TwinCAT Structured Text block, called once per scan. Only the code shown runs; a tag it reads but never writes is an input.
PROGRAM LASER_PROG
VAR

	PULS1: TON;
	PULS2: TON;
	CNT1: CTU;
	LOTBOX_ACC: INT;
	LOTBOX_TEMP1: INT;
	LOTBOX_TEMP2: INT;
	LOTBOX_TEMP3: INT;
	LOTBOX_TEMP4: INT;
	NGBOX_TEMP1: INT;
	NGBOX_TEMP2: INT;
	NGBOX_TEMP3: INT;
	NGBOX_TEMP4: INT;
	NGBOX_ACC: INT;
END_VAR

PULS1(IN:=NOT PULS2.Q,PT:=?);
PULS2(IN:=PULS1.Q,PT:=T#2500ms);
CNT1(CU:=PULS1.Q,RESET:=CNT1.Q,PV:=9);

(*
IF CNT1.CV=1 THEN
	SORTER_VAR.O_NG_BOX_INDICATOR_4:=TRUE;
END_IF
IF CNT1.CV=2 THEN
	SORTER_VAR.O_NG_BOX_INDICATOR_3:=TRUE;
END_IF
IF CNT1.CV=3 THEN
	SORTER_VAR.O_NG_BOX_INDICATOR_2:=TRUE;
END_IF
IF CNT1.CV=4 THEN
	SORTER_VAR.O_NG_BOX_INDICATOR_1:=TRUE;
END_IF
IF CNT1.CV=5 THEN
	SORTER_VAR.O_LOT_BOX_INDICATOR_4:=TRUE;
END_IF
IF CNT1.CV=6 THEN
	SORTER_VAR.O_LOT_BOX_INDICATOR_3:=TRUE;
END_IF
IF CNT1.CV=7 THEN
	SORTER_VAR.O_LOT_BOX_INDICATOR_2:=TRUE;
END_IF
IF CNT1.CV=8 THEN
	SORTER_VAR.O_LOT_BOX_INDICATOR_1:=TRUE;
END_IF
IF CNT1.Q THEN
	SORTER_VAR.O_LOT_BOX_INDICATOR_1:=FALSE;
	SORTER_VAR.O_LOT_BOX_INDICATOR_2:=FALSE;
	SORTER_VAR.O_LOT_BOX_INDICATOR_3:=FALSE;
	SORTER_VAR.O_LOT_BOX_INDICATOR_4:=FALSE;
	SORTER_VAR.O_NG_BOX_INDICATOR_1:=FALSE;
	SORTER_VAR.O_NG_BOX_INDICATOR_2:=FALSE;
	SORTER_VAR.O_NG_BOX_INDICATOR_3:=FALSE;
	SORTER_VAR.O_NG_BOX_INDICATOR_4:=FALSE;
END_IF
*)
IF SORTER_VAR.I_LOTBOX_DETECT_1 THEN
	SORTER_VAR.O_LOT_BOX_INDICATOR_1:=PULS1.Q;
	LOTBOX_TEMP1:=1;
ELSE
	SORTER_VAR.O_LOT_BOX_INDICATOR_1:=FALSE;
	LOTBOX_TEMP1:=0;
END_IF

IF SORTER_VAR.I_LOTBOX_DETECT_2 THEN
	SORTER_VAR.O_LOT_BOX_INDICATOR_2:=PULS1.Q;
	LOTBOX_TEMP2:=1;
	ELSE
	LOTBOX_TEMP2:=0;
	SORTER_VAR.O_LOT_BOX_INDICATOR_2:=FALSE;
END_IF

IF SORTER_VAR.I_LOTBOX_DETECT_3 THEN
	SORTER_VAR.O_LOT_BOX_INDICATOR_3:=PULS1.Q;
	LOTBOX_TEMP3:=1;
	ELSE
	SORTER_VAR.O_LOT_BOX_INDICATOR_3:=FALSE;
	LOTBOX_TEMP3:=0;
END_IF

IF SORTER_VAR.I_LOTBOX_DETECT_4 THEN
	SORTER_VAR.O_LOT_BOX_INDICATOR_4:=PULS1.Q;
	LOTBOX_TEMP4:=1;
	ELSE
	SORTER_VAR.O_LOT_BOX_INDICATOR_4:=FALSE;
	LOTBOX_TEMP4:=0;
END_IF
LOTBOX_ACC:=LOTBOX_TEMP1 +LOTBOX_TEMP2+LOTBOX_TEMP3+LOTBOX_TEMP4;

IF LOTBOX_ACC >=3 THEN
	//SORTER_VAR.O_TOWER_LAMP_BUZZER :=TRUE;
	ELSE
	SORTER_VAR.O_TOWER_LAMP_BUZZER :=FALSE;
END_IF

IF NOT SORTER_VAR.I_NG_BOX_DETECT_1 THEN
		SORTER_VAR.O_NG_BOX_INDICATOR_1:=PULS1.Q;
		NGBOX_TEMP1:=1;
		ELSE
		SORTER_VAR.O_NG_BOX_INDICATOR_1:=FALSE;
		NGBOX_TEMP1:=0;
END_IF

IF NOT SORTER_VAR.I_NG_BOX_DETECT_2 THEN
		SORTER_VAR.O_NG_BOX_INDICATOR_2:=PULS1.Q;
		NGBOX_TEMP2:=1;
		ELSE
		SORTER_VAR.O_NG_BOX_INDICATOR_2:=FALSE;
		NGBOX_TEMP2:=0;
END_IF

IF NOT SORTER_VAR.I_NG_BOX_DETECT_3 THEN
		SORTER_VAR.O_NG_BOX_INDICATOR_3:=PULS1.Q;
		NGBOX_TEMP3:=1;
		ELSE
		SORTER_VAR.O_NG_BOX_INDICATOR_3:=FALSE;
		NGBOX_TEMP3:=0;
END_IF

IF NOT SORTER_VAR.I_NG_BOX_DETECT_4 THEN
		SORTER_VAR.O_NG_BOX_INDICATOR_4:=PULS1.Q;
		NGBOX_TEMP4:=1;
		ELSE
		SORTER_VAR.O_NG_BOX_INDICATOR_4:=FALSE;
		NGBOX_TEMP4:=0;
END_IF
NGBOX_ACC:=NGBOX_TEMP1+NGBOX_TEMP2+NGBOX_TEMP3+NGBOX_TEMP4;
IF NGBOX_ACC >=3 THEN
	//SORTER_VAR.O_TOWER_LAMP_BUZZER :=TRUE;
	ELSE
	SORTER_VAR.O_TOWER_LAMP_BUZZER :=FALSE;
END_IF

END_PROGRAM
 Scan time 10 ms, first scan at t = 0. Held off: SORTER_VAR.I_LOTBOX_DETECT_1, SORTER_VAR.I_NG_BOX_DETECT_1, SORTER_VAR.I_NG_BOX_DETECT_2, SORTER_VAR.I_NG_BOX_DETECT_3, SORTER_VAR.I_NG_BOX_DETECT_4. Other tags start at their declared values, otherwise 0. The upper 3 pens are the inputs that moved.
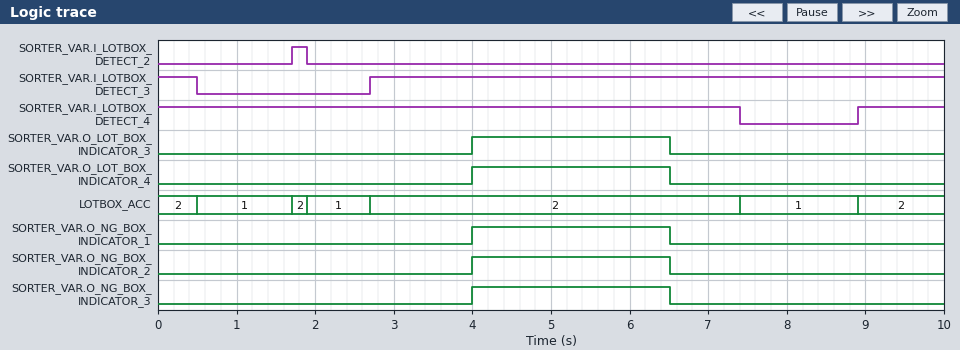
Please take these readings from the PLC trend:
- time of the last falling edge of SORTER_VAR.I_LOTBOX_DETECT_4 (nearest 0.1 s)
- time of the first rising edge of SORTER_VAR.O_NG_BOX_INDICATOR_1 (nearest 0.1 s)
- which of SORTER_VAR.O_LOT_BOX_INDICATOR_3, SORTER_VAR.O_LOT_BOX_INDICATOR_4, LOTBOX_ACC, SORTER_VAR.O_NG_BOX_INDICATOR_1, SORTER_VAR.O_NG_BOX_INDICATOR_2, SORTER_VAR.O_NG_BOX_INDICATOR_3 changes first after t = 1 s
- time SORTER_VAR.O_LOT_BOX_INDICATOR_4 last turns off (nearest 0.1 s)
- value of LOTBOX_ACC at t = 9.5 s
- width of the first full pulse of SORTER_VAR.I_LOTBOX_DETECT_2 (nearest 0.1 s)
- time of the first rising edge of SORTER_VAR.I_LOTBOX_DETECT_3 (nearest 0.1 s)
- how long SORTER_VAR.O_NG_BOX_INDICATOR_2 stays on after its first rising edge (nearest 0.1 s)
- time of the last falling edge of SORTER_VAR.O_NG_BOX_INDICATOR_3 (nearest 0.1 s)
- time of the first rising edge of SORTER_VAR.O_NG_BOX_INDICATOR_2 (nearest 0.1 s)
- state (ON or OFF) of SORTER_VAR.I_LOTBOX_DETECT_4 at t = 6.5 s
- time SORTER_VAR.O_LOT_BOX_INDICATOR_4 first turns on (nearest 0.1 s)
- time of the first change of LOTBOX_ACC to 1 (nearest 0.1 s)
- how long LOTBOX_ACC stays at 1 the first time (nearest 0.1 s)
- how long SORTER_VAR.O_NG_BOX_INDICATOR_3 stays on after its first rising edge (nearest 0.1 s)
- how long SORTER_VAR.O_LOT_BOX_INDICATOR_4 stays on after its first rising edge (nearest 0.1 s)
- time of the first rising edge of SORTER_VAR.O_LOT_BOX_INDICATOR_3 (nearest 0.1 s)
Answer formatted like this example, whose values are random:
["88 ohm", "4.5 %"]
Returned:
["7.4 s", "4.0 s", "LOTBOX_ACC", "6.5 s", "2", "0.2 s", "2.7 s", "2.5 s", "6.5 s", "4.0 s", "ON", "4.0 s", "0.5 s", "1.2 s", "2.5 s", "2.5 s", "4.0 s"]
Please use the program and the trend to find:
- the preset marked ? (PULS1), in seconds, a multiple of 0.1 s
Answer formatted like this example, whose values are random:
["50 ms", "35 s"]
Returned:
["4.0 s"]
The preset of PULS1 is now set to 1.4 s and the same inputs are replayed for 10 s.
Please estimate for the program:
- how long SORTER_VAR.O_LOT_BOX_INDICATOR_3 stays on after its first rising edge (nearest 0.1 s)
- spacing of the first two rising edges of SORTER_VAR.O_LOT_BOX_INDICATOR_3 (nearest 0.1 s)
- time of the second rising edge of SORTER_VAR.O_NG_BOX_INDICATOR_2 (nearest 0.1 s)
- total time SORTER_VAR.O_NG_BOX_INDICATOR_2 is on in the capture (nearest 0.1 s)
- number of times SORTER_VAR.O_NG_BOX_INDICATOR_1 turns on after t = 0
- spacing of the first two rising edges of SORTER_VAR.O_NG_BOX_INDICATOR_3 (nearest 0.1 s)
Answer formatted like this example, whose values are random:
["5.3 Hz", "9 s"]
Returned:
["1.2 s", "2.6 s", "5.3 s", "5.8 s", "3", "3.9 s"]
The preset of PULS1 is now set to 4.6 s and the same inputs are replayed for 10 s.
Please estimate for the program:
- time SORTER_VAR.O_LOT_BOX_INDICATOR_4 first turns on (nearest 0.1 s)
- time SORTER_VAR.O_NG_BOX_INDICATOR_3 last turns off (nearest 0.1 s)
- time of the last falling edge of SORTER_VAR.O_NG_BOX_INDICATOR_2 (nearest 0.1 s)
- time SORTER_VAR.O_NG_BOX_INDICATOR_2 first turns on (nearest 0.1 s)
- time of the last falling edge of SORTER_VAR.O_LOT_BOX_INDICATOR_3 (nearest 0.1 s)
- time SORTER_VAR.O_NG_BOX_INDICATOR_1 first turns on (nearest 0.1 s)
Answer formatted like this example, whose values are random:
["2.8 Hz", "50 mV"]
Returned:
["4.6 s", "7.1 s", "7.1 s", "4.6 s", "7.1 s", "4.6 s"]
